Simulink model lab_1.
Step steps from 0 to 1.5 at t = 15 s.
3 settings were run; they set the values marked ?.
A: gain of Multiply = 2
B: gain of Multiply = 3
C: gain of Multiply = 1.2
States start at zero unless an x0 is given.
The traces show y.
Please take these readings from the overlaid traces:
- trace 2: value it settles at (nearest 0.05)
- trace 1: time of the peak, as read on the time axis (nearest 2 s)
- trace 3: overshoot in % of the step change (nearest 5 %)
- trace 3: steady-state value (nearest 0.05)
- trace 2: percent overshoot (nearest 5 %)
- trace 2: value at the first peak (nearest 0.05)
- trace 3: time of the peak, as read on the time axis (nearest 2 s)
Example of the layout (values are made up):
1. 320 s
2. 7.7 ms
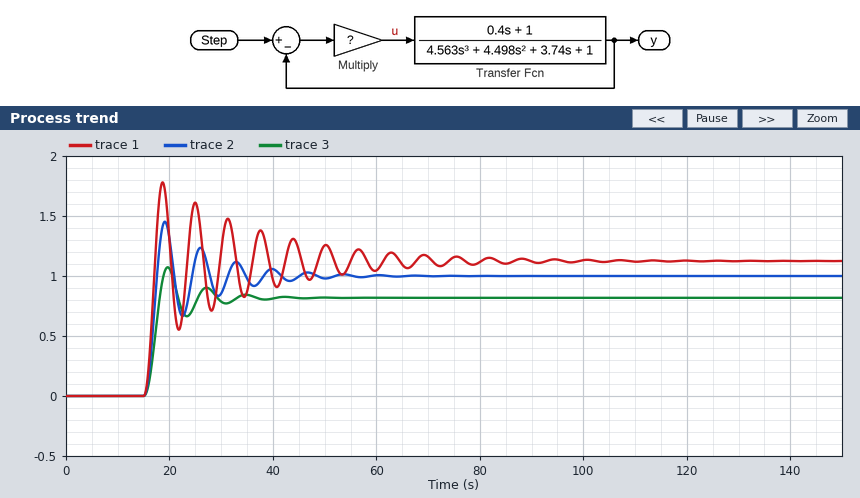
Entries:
1. 1.00
2. 18 s
3. 30 %
4. 0.80
5. 45 %
6. 1.45
7. 20 s
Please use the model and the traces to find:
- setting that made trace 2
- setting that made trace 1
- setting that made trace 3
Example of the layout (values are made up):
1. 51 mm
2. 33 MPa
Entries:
1. A
2. B
3. C
